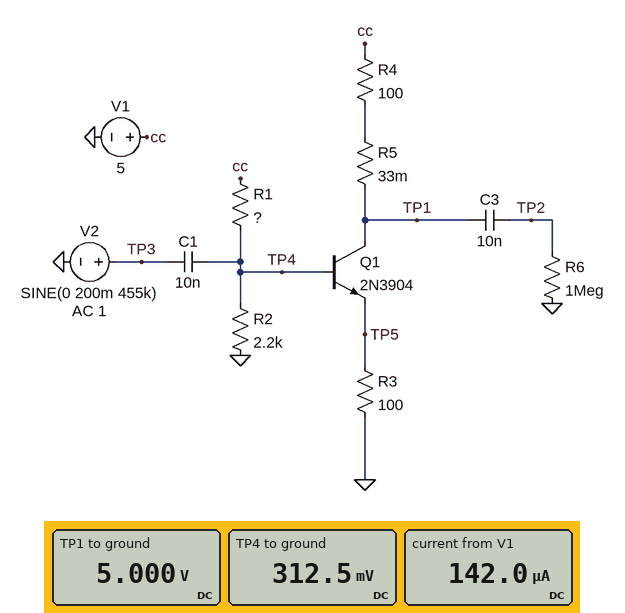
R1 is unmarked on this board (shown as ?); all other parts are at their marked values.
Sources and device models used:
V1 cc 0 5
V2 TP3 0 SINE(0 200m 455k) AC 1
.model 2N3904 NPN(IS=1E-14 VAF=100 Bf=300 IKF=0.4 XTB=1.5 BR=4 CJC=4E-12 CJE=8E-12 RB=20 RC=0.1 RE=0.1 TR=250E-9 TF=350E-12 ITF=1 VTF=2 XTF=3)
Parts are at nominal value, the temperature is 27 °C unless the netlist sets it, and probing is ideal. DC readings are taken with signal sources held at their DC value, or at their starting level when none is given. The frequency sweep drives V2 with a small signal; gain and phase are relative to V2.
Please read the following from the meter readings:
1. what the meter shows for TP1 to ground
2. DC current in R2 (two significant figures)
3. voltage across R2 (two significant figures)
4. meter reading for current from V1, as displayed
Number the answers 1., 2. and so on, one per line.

1. 5.000 V
2. 140 µA
3. 310 mV
4. 142.0 µA
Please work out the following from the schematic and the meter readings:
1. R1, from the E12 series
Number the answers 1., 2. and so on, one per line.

1. 33 kΩ
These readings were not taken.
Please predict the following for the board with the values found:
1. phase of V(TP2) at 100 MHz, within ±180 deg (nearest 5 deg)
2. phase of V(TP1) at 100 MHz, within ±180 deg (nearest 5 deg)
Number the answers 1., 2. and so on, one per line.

1. 75 deg
2. 75 deg
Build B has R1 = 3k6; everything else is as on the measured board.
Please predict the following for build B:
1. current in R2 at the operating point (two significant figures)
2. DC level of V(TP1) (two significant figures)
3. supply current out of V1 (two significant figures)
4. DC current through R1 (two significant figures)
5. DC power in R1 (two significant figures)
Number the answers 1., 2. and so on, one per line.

1. 840 µA
2. 3.9 V
3. 12 mA
4. 880 µA
5. 2.8 mW
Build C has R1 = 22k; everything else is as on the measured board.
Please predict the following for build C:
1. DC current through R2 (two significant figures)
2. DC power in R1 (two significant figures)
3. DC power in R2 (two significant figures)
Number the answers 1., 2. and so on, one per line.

1. 210 µA
2. 940 µW
3. 94 µW
